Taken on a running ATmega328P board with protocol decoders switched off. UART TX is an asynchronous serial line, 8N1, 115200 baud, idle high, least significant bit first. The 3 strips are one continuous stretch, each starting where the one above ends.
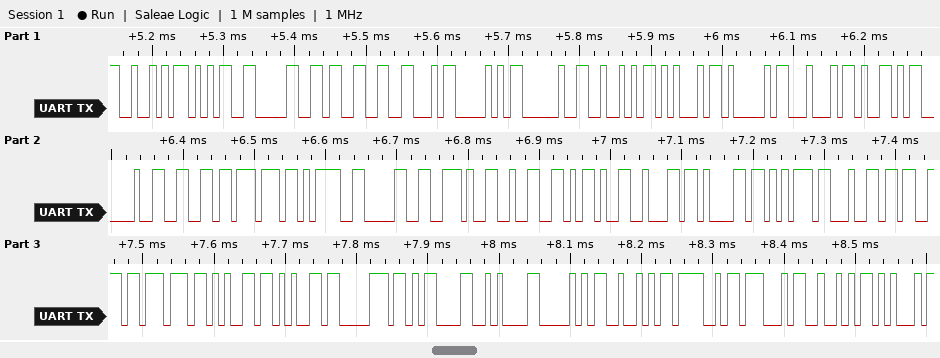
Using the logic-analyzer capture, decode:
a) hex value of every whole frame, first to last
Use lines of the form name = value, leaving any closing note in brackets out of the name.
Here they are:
hex value of every whole frame, first to last = 52 35 30 33 46 50 20 52 45 41 44 59 20 66 77 3D 30 2E 32 2D 62 61 75 64 73 77 65 65 70 0D 0A 50 52 4F 47 52 45
